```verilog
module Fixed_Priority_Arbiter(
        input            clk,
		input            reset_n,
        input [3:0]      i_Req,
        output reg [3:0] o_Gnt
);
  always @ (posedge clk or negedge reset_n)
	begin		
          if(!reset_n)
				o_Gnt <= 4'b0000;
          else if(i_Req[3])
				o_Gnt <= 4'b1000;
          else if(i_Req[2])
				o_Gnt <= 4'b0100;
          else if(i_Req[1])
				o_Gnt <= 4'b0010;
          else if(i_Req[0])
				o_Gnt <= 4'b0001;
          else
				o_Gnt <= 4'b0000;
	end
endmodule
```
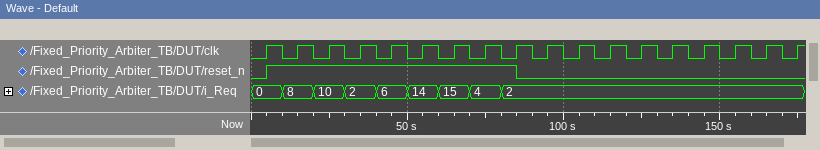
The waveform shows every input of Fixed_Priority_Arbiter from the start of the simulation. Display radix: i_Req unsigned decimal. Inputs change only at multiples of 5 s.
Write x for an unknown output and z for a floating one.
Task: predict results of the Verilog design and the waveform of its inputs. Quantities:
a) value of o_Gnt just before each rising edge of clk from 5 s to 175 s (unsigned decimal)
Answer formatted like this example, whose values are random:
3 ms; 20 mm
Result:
0, 0, 8, 8, 2, 4, 8, 8, 4, 0, 0, 0, 0, 0, 0, 0, 0, 0
